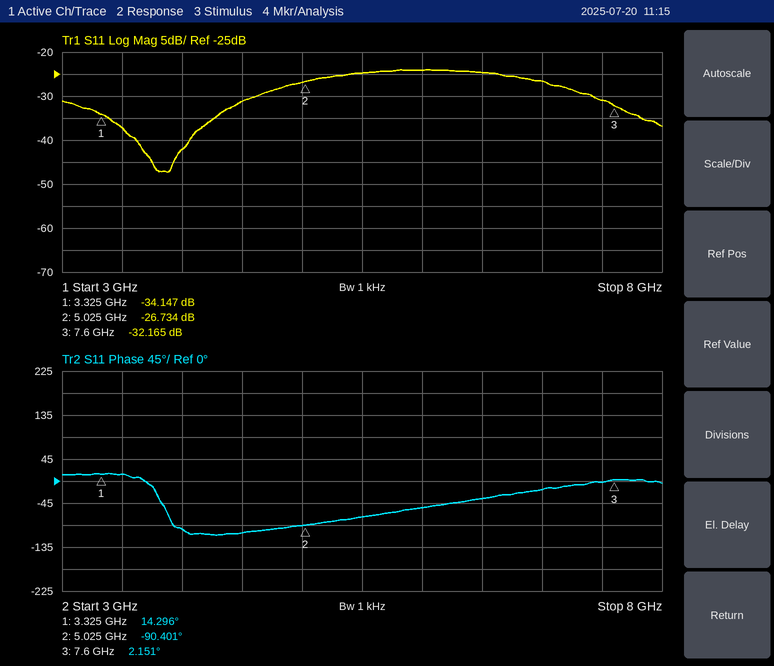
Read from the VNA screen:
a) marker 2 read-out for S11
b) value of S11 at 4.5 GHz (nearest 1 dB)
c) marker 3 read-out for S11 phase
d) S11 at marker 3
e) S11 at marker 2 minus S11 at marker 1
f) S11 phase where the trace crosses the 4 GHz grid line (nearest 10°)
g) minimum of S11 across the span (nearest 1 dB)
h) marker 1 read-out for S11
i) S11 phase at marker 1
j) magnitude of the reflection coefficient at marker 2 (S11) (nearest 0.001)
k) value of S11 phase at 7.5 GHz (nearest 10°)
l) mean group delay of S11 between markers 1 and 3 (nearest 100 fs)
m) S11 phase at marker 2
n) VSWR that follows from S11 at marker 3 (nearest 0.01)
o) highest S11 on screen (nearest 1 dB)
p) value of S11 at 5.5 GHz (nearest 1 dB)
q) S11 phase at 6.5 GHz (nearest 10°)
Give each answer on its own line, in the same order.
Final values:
-26.734 dB
-31 dB
2.151°
-32.165 dB
7.413 dB
-100°
-47 dB
-34.147 dB
14.296°
0.046
0°
7.9 ps
-90.401°
1.05
-24 dB
-25 dB
-40°
